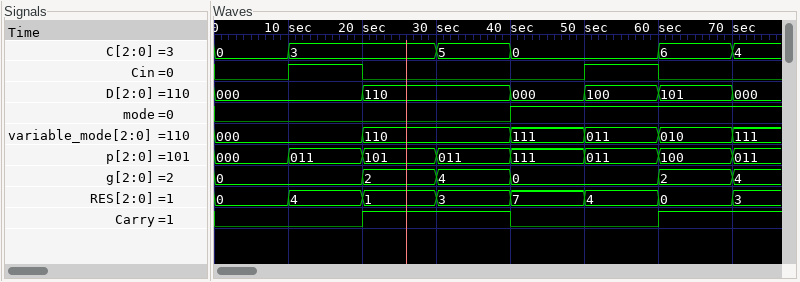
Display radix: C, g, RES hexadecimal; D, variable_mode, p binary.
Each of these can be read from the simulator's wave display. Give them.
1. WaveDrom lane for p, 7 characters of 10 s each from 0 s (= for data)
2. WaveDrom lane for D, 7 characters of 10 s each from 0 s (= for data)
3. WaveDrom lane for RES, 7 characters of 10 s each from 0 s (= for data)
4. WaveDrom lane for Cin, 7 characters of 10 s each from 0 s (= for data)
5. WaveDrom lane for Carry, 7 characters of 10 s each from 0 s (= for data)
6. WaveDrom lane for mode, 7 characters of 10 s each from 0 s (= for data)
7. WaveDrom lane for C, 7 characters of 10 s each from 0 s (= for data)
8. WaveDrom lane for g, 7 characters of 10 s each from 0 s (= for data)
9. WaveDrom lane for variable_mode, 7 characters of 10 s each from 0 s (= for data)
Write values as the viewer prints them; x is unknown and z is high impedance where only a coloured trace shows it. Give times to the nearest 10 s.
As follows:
{name: 'p', wave: '=======', data: '000 011 101 011 111 011 100'}
{name: 'D', wave: '=.=.===', data: '000 110 000 100 101'}
{name: 'RES', wave: '=======', data: '0 4 1 3 7 4 0'}
{name: 'Cin', wave: '010..10'}
{name: 'Carry', wave: '0.1.0.1'}
{name: 'mode', wave: '0...1..'}
{name: 'C', wave: '==.==.=', data: '0 3 5 0 6'}
{name: 'g', wave: '=.===.=', data: '0 2 4 0 2'}
{name: 'variable_mode', wave: '=.=.===', data: '000 110 111 011 010'}
